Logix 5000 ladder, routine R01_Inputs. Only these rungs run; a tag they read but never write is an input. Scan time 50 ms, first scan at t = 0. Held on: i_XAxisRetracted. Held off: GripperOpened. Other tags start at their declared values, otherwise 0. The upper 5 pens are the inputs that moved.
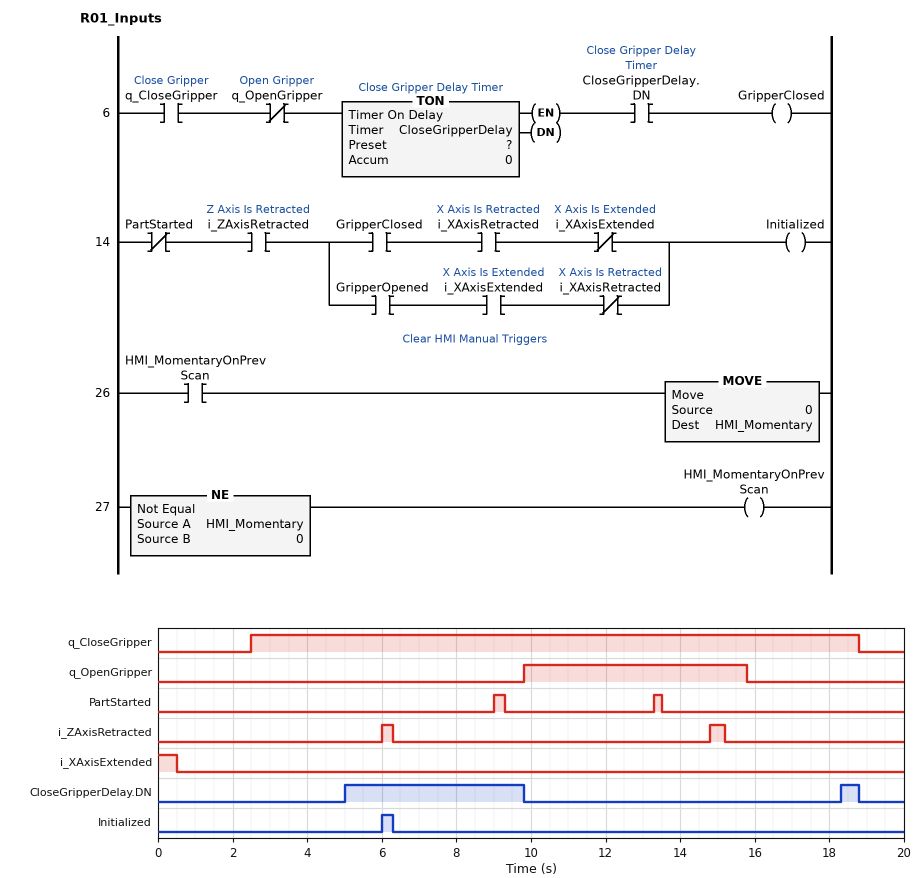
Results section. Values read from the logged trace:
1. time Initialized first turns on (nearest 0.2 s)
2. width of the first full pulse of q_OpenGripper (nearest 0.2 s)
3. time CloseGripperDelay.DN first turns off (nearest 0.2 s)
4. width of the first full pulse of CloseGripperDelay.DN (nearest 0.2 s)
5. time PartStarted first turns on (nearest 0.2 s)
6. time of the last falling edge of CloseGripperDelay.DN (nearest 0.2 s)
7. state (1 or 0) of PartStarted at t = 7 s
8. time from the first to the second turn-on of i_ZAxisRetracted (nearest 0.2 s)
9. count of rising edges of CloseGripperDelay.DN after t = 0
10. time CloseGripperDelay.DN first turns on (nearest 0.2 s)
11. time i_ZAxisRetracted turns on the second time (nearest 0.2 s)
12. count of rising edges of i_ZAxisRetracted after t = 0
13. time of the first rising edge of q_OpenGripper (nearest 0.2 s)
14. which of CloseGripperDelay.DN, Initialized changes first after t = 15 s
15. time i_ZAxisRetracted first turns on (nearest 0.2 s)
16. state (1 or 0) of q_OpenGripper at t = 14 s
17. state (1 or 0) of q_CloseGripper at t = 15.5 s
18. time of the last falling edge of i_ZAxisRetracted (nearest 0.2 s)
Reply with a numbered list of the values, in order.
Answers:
1. 6.0 s
2. 6.0 s
3. 9.8 s
4. 4.8 s
5. 9.0 s
6. 18.8 s
7. 0
8. 8.8 s
9. 2
10. 5.0 s
11. 14.8 s
12. 2
13. 9.8 s
14. CloseGripperDelay.DN
15. 6.0 s
16. 1
17. 1
18. 15.2 s
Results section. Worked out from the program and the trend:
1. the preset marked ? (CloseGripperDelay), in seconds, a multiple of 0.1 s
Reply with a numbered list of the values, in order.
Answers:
1. 2.5 s
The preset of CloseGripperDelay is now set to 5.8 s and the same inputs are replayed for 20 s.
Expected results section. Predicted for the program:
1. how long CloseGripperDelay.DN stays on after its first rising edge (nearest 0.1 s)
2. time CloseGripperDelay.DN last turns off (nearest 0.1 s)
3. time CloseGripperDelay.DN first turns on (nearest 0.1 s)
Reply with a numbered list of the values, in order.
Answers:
1. 1.5 s
2. 9.8 s
3. 8.3 s
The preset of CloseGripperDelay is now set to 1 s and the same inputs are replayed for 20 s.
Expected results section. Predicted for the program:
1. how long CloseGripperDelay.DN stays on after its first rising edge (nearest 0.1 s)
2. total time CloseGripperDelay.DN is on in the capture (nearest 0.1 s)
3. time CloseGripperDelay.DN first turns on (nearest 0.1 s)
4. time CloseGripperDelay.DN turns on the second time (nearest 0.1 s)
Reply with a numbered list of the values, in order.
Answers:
1. 6.3 s
2. 8.3 s
3. 3.5 s
4. 16.8 s
